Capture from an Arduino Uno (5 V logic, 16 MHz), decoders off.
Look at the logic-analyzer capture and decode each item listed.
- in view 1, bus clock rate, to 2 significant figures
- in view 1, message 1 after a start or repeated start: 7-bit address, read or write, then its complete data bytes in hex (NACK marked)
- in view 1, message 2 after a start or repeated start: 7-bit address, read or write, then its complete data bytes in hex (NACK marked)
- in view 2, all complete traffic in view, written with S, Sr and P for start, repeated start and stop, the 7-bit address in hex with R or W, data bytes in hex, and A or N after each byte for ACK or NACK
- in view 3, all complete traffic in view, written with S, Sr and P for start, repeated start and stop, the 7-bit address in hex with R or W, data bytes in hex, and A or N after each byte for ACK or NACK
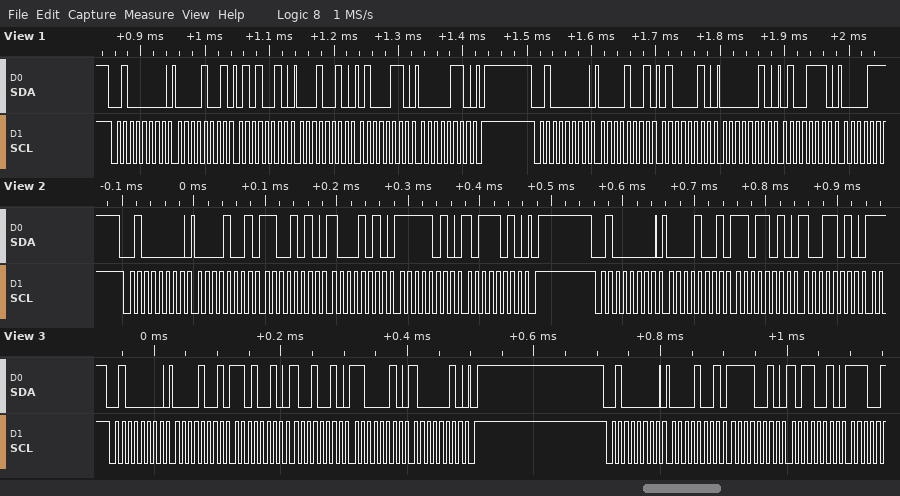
100 kHz
0x20 write: 09 52 12 46 06
0x20 write: 09 42 02 4E
S 20W A 09 A CA A 8A A FA A BA A P S 20W A 09 A DA A 9A A
S 20W A 09 A D2 A 92 A C2 A 82 A P S 20W A 09 A F2 A B2 A
